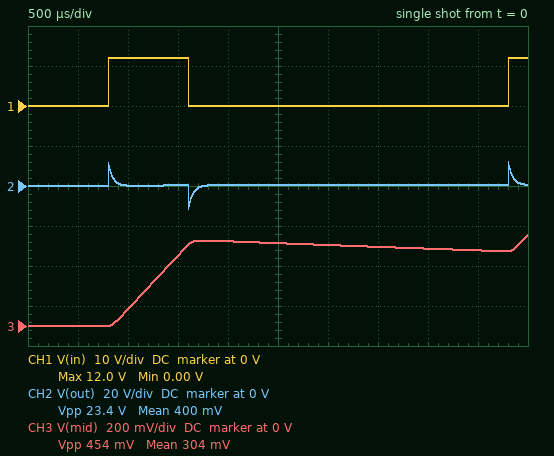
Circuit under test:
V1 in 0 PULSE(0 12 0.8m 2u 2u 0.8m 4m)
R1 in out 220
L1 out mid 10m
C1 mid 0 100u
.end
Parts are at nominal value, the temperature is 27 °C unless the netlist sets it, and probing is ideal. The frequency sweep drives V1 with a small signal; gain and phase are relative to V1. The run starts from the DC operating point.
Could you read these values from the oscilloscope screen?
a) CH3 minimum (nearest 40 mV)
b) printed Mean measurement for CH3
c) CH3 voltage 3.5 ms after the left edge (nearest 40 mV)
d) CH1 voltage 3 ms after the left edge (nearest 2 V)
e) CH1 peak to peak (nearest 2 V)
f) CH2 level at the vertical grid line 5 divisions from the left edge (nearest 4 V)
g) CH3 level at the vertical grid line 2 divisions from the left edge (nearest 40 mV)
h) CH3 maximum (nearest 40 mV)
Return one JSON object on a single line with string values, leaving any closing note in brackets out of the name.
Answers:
{"CH3 minimum": "0 V", "printed Mean measurement for CH3": "304 mV", "CH3 voltage 3.5 ms after the left edge": "400 mV", "CH1 voltage 3 ms after the left edge": "0 V", "CH1 peak to peak": "12 V", "CH2 level at the vertical grid line 5 divisions from the left edge": "0 V", "CH3 level at the vertical grid line 2 divisions from the left edge": "80 mV", "CH3 maximum": "440 mV"}
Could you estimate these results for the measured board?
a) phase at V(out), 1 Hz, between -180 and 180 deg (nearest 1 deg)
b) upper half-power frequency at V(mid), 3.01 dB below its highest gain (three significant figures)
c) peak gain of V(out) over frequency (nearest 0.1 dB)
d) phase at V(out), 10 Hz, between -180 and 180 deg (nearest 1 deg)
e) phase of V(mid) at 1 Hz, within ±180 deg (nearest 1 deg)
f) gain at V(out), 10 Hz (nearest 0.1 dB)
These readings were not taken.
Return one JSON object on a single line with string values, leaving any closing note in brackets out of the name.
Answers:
{"phase at V(out), 1 Hz, between -180 and 180 deg": "-8 deg", "upper half-power frequency at V(mid), 3.01 dB below its highest gain": "7.25 Hz", "peak gain of V(out) over frequency": "0 dB", "phase at V(out), 10 Hz, between -180 and 180 deg": "-54 deg", "phase of V(mid) at 1 Hz, within ±180 deg": "-8 deg", "gain at V(out), 10 Hz": "-4.7 dB"}
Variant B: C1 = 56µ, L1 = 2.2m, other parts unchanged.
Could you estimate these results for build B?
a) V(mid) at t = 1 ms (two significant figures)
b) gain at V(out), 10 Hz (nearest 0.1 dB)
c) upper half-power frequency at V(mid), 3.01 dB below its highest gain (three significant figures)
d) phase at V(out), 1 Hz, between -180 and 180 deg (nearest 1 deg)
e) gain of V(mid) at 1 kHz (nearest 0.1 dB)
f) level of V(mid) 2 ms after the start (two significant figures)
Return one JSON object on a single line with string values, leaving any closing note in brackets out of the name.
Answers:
{"V(mid) at t = 1 ms": "180 mV", "gain at V(out), 10 Hz": "-2.0 dB", "upper half-power frequency at V(mid), 3.01 dB below its highest gain": "12.9 Hz", "phase at V(out), 1 Hz, between -180 and 180 deg": "-4 deg", "gain of V(mid) at 1 kHz": "-37.8 dB", "level of V(mid) 2 ms after the start": "730 mV"}
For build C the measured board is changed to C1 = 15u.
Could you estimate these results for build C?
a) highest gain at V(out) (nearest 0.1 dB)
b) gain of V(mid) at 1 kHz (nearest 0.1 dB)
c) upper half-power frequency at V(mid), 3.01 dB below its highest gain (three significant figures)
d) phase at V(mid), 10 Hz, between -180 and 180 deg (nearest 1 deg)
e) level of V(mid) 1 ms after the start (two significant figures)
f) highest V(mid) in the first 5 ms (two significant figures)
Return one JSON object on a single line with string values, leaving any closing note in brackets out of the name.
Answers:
{"highest gain at V(out)": "0 dB", "gain of V(mid) at 1 kHz": "-26.6 dB", "upper half-power frequency at V(mid), 3.01 dB below its highest gain": "48.9 Hz", "phase at V(mid), 10 Hz, between -180 and 180 deg": "-12 deg", "level of V(mid) 1 ms after the start": "550 mV", "highest V(mid) in the first 5 ms": "2.6 V"}
